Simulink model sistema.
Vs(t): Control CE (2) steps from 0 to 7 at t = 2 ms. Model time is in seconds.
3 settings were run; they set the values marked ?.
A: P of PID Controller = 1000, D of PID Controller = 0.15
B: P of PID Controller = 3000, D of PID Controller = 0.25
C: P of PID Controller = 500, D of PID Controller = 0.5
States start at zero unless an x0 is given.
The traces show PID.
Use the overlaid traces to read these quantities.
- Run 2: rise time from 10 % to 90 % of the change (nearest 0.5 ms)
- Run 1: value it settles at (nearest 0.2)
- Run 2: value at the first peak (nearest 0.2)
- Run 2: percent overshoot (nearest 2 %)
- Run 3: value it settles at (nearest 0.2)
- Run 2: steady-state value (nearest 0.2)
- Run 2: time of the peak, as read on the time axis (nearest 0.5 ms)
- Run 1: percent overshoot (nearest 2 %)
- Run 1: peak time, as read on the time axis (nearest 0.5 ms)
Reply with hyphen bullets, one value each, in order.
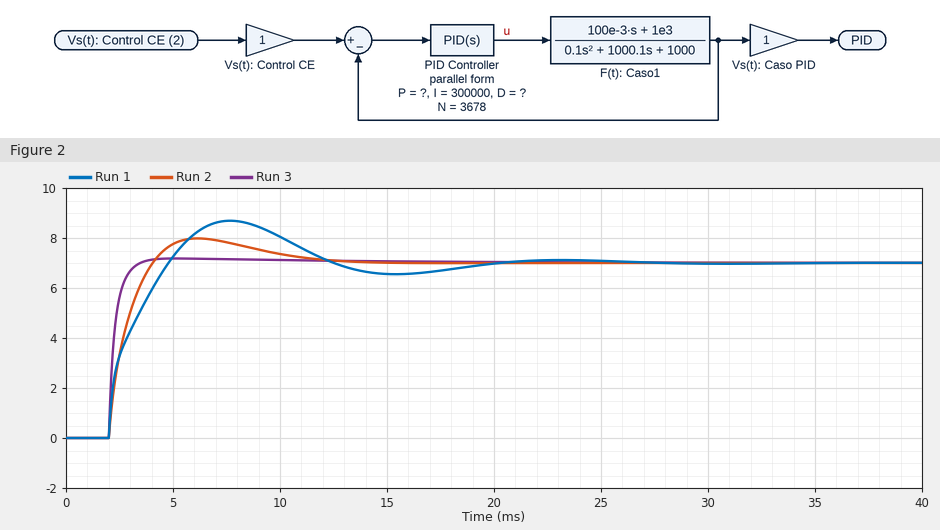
- 1.5 ms
- 7.0
- 8.0
- 14 %
- 7.0
- 7.0
- 6.0 ms
- 24 %
- 7.5 ms
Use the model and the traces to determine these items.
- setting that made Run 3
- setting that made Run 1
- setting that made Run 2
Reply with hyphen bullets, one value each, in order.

- B
- C
- A
